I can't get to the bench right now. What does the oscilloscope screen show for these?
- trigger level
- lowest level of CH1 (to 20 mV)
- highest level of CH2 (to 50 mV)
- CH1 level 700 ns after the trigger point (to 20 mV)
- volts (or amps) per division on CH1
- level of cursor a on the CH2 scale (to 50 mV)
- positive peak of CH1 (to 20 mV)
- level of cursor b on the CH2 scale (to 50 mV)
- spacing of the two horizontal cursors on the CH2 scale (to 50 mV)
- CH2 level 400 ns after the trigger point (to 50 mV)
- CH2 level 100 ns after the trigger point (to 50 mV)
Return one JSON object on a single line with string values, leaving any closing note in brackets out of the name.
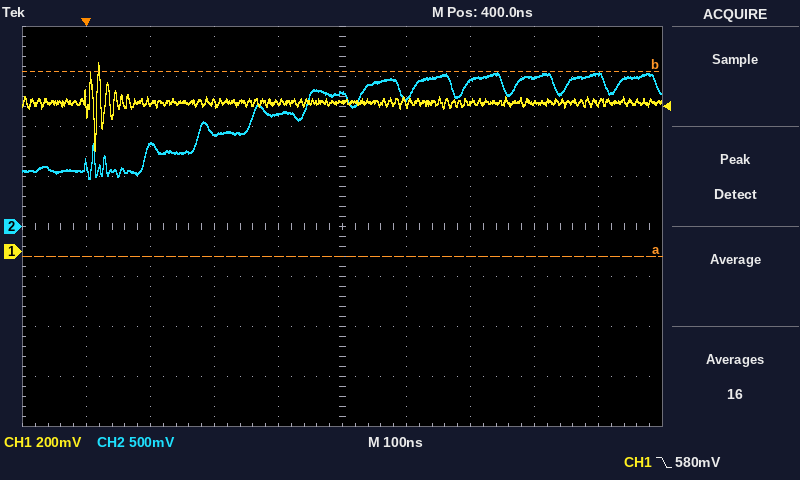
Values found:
{"trigger level": "580 mV", "lowest level of CH1": "400 mV", "highest level of CH2": "1.55 V", "CH1 level 700 ns after the trigger point": "600 mV", "volts (or amps) per division on CH1": "200 mV", "level of cursor a on the CH2 scale": "-300 mV", "positive peak of CH1": "760 mV", "level of cursor b on the CH2 scale": "1.55 V", "spacing of the two horizontal cursors on the CH2 scale": "1.85 V", "CH2 level 400 ns after the trigger point": "1.35 V", "CH2 level 100 ns after the trigger point": "800 mV"}
